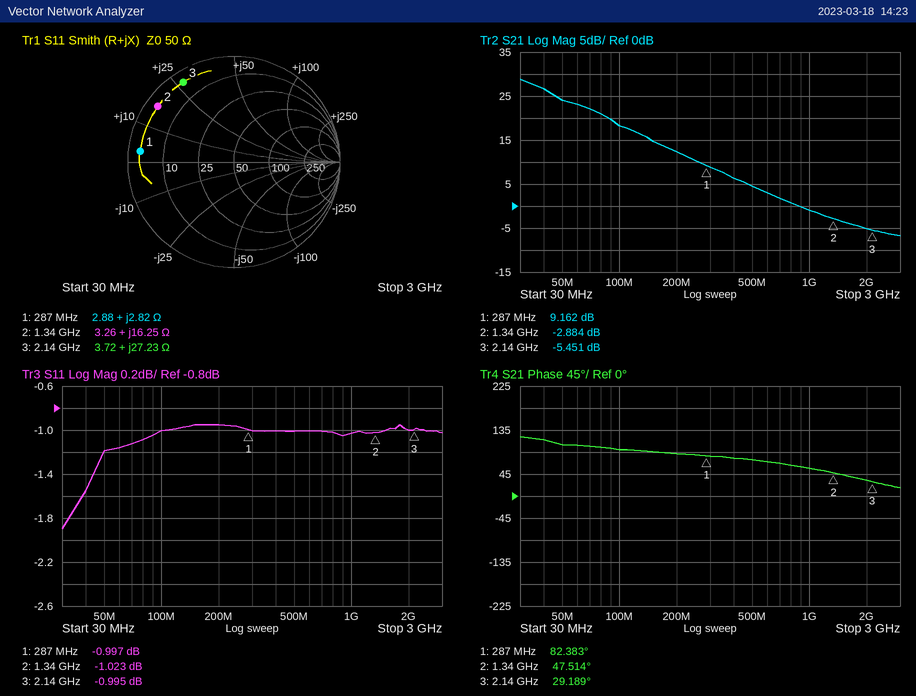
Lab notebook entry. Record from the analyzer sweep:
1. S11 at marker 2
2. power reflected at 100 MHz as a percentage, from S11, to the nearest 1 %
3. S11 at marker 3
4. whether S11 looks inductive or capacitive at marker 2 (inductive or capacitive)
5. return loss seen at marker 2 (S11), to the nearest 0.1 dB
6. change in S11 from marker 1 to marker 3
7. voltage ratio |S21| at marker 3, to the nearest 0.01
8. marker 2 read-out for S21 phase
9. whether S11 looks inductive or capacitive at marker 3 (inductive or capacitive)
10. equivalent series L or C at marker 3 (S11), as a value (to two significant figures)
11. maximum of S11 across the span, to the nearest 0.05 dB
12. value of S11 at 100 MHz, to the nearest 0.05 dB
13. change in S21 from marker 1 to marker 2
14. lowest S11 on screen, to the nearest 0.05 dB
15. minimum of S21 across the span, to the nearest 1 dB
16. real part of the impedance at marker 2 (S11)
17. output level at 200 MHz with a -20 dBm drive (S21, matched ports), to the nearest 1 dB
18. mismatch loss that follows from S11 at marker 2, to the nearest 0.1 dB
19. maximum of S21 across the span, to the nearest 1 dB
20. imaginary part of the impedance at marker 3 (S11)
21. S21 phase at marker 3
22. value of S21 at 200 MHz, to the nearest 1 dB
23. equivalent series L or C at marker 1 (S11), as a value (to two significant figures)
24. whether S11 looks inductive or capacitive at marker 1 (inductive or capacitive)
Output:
-1.023 dB
79 %
-0.995 dB
inductive
1.0 dB
0.002 dB
0.53
47.514°
inductive
2.0 nH
-0.95 dB
-1.00 dB
-12.046 dB
-1.90 dB
-7 dB
3.26 Ω
-8 dBm
6.8 dB
29 dB
+27.23 Ω
29.189°
12 dB
1.6 nH
inductive
